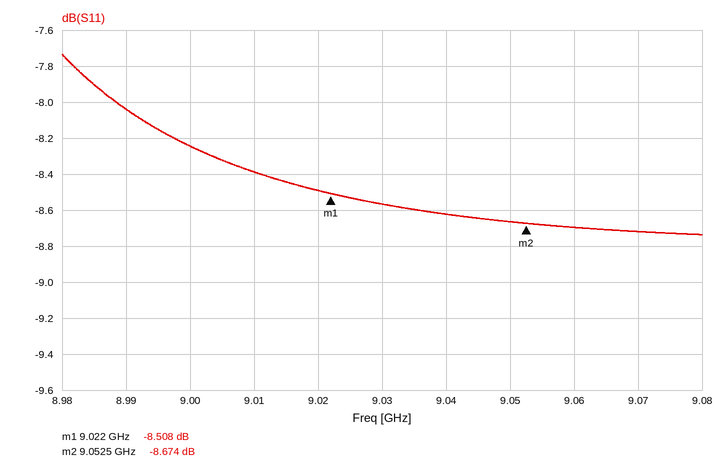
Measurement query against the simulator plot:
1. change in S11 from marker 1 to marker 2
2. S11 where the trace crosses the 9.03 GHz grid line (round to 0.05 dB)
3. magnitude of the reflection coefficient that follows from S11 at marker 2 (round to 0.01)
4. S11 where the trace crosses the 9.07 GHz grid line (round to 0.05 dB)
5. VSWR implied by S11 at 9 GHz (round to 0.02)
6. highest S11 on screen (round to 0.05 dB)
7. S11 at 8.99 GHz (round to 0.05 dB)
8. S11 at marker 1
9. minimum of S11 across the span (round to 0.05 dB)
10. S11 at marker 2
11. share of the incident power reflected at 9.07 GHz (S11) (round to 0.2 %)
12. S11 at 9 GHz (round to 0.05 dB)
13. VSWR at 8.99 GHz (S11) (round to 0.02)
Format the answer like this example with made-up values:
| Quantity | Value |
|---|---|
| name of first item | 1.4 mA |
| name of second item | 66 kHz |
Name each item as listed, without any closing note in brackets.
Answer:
| Quantity | Value |
|---|---|
| change in S11 from marker 1 to marker 2 | -0.166 dB |
| S11 where the trace crosses the 9.03 GHz grid line | -8.55 dB |
| magnitude of the reflection coefficient that follows from S11 at marker 2 | 0.37 |
| S11 where the trace crosses the 9.07 GHz grid line | -8.70 dB |
| VSWR implied by S11 at 9 GHz | 2.26 |
| highest S11 on screen | -7.75 dB |
| S11 at 8.99 GHz | -8.05 dB |
| S11 at marker 1 | -8.508 dB |
| minimum of S11 across the span | -8.75 dB |
| S11 at marker 2 | -8.674 dB |
| share of the incident power reflected at 9.07 GHz (S11) | 13.4 % |
| S11 at 9 GHz | -8.25 dB |
| VSWR at 8.99 GHz (S11) | 2.32 |
